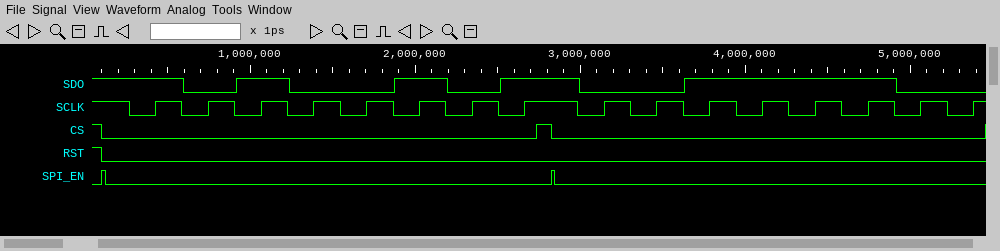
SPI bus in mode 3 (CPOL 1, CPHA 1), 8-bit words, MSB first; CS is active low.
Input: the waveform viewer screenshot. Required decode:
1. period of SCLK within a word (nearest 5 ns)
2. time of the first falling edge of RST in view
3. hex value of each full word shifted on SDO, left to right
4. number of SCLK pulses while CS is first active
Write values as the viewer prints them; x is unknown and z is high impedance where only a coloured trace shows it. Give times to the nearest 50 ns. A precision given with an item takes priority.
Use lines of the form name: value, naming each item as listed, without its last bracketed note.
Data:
period of SCLK within a word: 320 ns
time of the first falling edge of RST in view: 100 ns
hex value of each full word shifted on SDO, left to right: A5, 3C
number of SCLK pulses while CS is first active: 8
